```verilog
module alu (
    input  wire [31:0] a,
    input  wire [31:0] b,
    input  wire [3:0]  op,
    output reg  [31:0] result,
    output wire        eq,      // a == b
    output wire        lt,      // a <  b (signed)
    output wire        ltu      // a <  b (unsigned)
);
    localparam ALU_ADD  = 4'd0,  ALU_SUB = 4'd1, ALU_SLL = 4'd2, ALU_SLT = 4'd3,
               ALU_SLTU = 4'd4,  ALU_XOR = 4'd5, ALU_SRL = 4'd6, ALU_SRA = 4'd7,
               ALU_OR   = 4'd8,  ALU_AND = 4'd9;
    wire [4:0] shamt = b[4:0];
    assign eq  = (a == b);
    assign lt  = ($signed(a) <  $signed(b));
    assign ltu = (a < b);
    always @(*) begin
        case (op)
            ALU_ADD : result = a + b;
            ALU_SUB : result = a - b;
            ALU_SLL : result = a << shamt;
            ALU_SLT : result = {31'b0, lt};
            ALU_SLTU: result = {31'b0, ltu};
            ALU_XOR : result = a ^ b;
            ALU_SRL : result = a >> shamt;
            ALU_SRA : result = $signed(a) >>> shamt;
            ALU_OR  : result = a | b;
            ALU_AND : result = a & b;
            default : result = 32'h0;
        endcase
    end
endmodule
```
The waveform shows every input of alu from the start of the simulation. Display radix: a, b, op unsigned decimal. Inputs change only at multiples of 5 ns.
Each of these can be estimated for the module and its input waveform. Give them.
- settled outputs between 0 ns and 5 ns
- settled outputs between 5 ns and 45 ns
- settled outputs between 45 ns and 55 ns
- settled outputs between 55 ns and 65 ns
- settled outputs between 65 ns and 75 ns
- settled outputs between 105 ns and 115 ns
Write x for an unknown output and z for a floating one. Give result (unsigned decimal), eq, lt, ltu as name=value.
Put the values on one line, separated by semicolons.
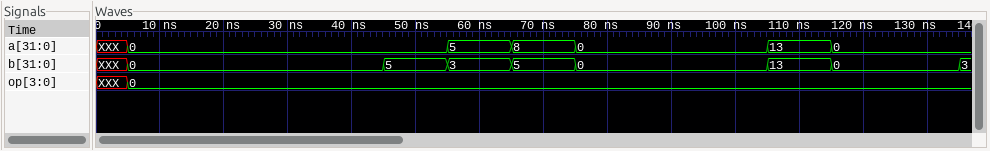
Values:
result=x, eq=x, lt=x, ltu=x; result=0, eq=1, lt=0, ltu=0; result=5, eq=0, lt=1, ltu=1; result=8, eq=0, lt=0, ltu=0; result=13, eq=0, lt=0, ltu=0; result=26, eq=1, lt=0, ltu=0
